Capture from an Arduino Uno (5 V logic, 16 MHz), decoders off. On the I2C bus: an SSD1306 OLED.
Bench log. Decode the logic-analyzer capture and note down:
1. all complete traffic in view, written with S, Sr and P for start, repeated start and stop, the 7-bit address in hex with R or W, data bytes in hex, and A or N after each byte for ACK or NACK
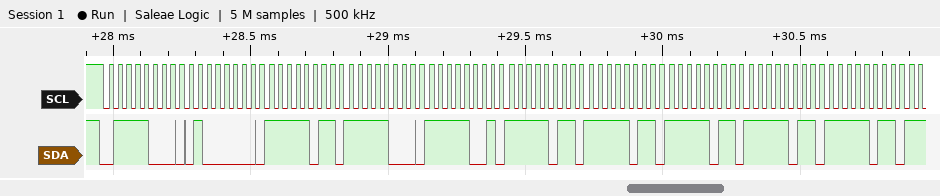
S 3CW A 40 A FB A F8 A F9 A FB A FB A FB A FB A FB A
